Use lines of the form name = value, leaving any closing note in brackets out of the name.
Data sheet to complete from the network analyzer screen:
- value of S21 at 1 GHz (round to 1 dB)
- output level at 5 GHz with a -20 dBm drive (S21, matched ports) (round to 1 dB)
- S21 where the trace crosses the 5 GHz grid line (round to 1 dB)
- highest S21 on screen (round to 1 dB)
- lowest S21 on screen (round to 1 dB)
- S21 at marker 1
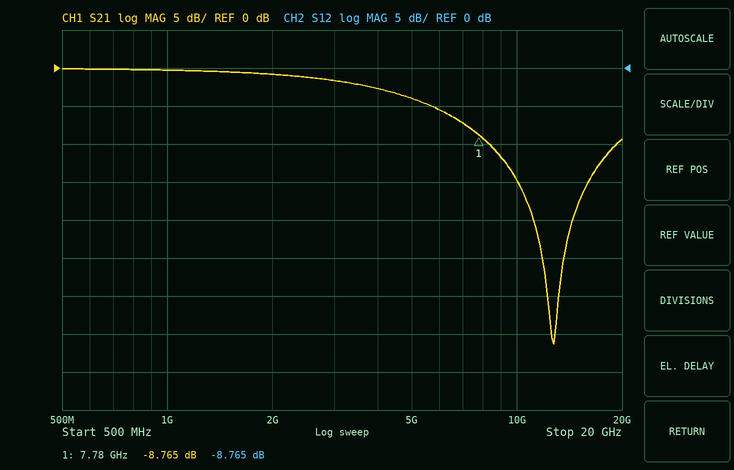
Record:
value of S21 at 1 GHz = 0 dB
output level at 5 GHz with a -20 dBm drive (S21, matched ports) = -24 dBm
S21 where the trace crosses the 5 GHz grid line = -4 dB
highest S21 on screen = 0 dB
lowest S21 on screen = -36 dB
S21 at marker 1 = -8.765 dB
